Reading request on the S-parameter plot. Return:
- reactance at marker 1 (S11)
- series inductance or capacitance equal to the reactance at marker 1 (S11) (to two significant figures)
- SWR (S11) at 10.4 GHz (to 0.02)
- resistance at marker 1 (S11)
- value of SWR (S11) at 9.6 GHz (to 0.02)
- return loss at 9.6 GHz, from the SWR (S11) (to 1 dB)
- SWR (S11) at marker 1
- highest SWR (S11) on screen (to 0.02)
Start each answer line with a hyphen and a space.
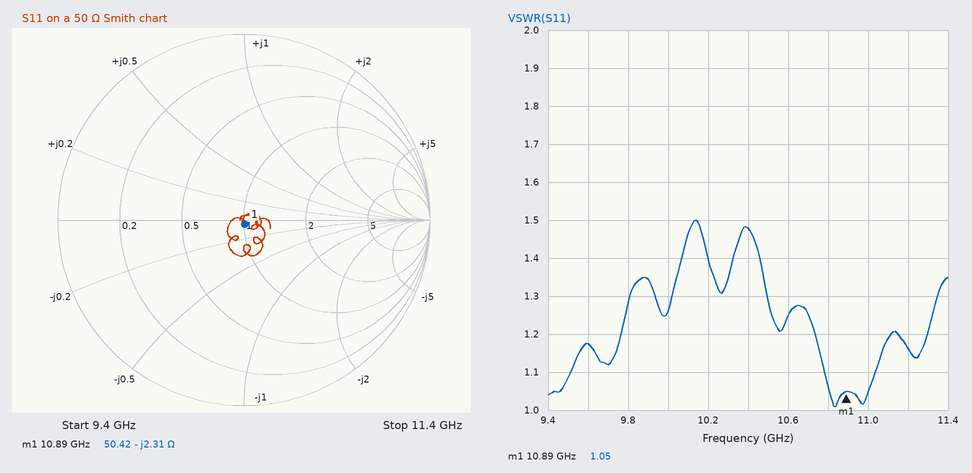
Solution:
- -2.31 Ω
- 6.3 pF
- 1.48
- 50.42 Ω
- 1.18
- 22 dB
- 1.05
- 1.50
